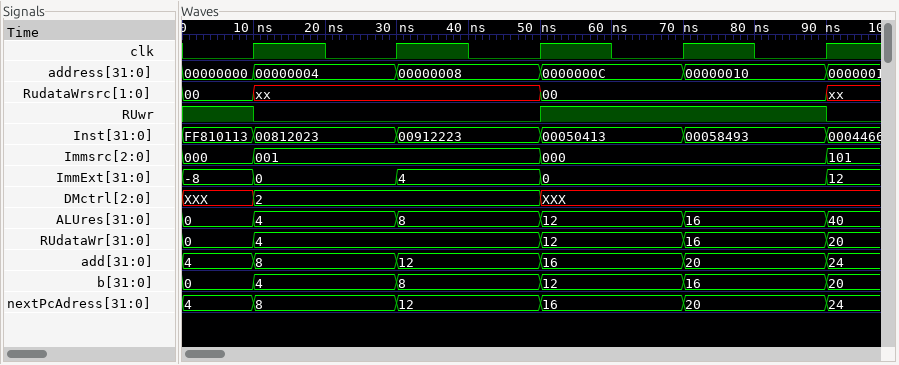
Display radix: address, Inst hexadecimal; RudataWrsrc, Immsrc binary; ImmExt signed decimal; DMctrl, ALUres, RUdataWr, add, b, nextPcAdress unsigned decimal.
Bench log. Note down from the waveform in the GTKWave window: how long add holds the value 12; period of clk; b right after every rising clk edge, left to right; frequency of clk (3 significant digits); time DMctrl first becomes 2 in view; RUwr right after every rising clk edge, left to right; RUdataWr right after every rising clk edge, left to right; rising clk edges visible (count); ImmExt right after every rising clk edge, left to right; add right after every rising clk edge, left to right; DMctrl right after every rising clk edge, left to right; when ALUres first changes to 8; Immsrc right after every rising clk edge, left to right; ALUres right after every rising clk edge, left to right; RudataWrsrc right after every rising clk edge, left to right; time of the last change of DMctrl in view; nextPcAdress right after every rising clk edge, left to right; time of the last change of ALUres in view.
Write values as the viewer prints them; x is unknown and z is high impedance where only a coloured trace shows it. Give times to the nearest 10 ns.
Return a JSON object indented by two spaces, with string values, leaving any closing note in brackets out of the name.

{
  "how long add holds the value 12": "20 ns",
  "period of clk": "20 ns",
  "b right after every rising clk edge, left to right": "4, 8, 12, 16, 20",
  "frequency of clk": "50.0 MHz",
  "time DMctrl first becomes 2 in view": "10 ns",
  "RUwr right after every rising clk edge, left to right": "0 0 1 1 0",
  "RUdataWr right after every rising clk edge, left to right": "4, 4, 12, 16, 20",
  "rising clk edges visible": "5",
  "ImmExt right after every rising clk edge, left to right": "0, 4, 0, 0, 12",
  "add right after every rising clk edge, left to right": "8, 12, 16, 20, 24",
  "DMctrl right after every rising clk edge, left to right": "2, 2, XXX, XXX, XXX",
  "when ALUres first changes to 8": "30 ns",
  "Immsrc right after every rising clk edge, left to right": "001, 001, 000, 000, 101",
  "ALUres right after every rising clk edge, left to right": "4, 8, 12, 16, 40",
  "RudataWrsrc right after every rising clk edge, left to right": "xx, xx, 00, 00, xx",
  "time of the last change of DMctrl in view": "50 ns",
  "nextPcAdress right after every rising clk edge, left to right": "8, 12, 16, 20, 24",
  "time of the last change of ALUres in view": "90 ns"
}
